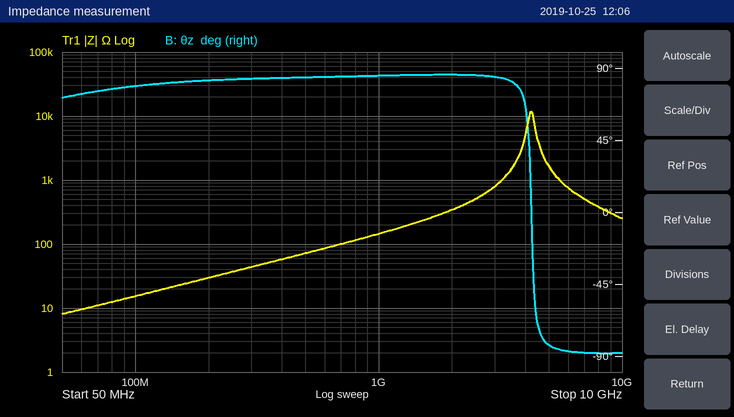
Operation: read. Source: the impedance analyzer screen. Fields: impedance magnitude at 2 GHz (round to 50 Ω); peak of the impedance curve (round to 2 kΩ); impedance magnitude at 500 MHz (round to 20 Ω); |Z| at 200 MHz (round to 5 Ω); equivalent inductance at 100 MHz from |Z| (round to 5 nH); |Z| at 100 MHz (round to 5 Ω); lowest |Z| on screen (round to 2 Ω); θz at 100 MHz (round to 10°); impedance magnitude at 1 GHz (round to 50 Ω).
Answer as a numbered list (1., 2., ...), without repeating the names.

1. 350 Ω
2. 12 kΩ
3. 80 Ω
4. 30 Ω
5. 25 nH
6. 15 Ω
7. 8 Ω
8. 80°
9. 150 Ω
